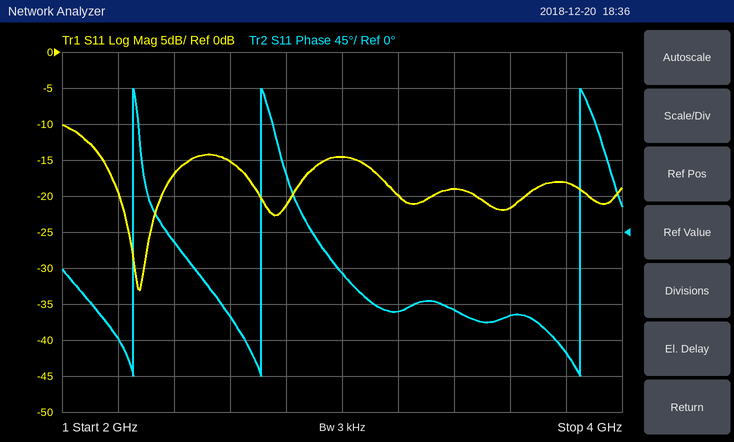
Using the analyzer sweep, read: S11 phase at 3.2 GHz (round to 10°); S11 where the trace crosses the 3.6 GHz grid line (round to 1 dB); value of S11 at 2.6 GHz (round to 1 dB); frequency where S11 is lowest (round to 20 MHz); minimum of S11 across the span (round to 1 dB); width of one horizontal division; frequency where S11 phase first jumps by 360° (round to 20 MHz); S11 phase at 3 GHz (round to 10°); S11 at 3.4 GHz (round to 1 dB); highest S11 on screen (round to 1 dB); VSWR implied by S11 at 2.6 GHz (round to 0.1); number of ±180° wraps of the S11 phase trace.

-100°
-22 dB
-15 dB
2.28 GHz
-33 dB
200 MHz
2.26 GHz
-50°
-19 dB
-10 dB
1.4
3
